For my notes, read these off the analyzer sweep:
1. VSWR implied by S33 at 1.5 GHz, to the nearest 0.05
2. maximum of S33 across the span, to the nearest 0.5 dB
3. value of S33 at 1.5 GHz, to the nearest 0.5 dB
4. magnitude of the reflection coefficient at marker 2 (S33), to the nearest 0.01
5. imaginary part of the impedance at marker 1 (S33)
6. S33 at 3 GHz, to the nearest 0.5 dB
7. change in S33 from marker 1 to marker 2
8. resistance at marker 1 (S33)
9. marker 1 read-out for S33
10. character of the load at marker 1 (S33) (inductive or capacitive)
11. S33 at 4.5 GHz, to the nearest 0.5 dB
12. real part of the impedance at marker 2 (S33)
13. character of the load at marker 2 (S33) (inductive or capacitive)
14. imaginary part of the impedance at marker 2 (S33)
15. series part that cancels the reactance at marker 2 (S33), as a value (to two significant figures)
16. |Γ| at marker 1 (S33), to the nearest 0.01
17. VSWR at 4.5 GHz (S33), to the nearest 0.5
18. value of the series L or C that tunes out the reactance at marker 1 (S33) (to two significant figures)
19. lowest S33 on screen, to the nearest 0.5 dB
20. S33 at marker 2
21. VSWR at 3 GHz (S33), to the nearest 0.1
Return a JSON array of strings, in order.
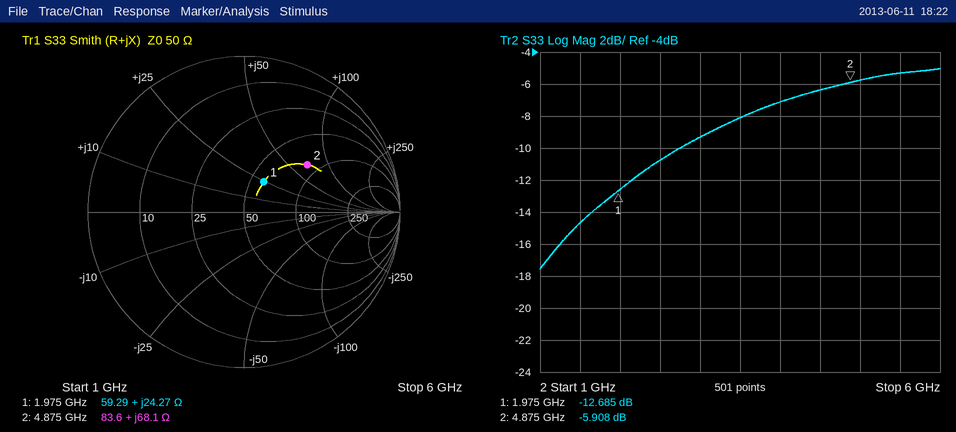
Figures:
["1.45", "-5.0 dB", "-14.5 dB", "0.51", "+24.27 Ω", "-9.5 dB", "6.777 dB", "59.29 Ω", "-12.685 dB", "inductive", "-6.5 dB", "83.6 Ω", "inductive", "+68.1 Ω", "480 fF", "0.23", "3.0", "3.3 pF", "-17.5 dB", "-5.908 dB", "2.0"]
